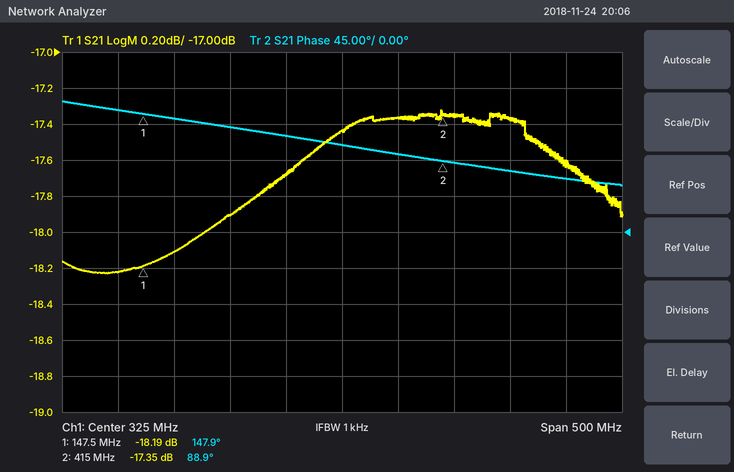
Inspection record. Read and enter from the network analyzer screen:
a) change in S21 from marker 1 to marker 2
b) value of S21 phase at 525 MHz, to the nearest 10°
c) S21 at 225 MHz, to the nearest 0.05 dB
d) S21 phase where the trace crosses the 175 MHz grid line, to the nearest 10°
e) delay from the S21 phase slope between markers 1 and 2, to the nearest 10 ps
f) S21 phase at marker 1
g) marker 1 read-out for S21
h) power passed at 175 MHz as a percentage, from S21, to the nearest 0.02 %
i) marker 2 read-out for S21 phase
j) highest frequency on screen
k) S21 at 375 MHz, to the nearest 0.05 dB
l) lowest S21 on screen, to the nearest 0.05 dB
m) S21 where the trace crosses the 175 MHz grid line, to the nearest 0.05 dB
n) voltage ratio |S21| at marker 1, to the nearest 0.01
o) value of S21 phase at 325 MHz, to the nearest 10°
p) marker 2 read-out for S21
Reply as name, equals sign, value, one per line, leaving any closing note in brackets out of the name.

change in S21 from marker 1 to marker 2 = 0.84 dB
value of S21 phase at 525 MHz, to the nearest 10° = 70°
S21 at 225 MHz, to the nearest 0.05 dB = -17.90 dB
S21 phase where the trace crosses the 175 MHz grid line, to the nearest 10° = 140°
delay from the S21 phase slope between markers 1 and 2, to the nearest 10 ps = 610 ps
S21 phase at marker 1 = 147.9°
marker 1 read-out for S21 = -18.19 dB
power passed at 175 MHz as a percentage, from S21, to the nearest 0.02 % = 1.54 %
marker 2 read-out for S21 phase = 88.9°
highest frequency on screen = 575 MHz
S21 at 375 MHz, to the nearest 0.05 dB = -17.35 dB
lowest S21 on screen, to the nearest 0.05 dB = -18.25 dB
S21 where the trace crosses the 175 MHz grid line, to the nearest 0.05 dB = -18.10 dB
voltage ratio |S21| at marker 1, to the nearest 0.01 = 0.12
value of S21 phase at 325 MHz, to the nearest 10° = 110°
marker 2 read-out for S21 = -17.35 dB
